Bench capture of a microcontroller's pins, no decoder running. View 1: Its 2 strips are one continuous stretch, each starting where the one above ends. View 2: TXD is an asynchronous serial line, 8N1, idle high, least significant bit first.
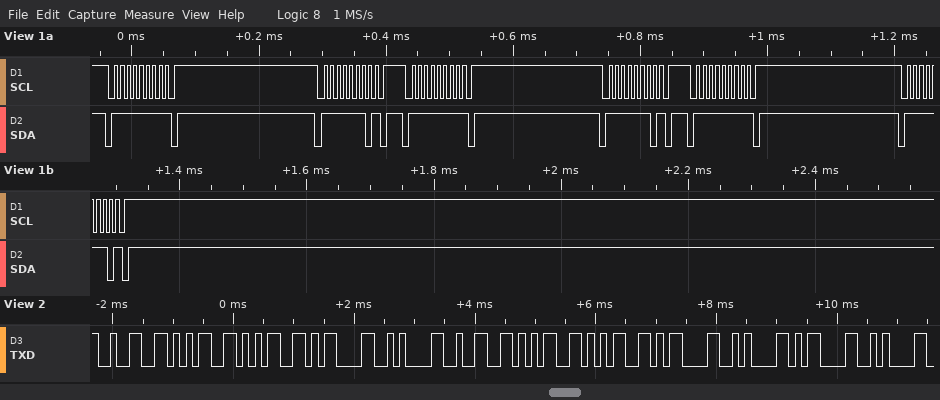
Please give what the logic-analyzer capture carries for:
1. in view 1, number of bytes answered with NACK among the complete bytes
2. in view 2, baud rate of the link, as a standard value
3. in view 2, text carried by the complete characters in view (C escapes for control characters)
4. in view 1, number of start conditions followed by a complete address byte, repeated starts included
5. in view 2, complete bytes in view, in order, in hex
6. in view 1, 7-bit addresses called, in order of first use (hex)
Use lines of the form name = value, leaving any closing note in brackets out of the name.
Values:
in view 1, number of bytes answered with NACK among the complete bytes = 6
in view 2, baud rate of the link, as a standard value = 9600 baud
in view 2, text carried by the complete characters in view = "255\r\n255\r\n\r\n"
in view 1, number of start conditions followed by a complete address byte, repeated starts included = 6
in view 2, complete bytes in view, in order, in hex = 0x32 0x35 0x35 0x0D 0x0A 0x32 0x35 0x35 0x0D 0x0A 0x0D 0x0A
in view 1, 7-bit addresses called, in order of first use = 0x7F
